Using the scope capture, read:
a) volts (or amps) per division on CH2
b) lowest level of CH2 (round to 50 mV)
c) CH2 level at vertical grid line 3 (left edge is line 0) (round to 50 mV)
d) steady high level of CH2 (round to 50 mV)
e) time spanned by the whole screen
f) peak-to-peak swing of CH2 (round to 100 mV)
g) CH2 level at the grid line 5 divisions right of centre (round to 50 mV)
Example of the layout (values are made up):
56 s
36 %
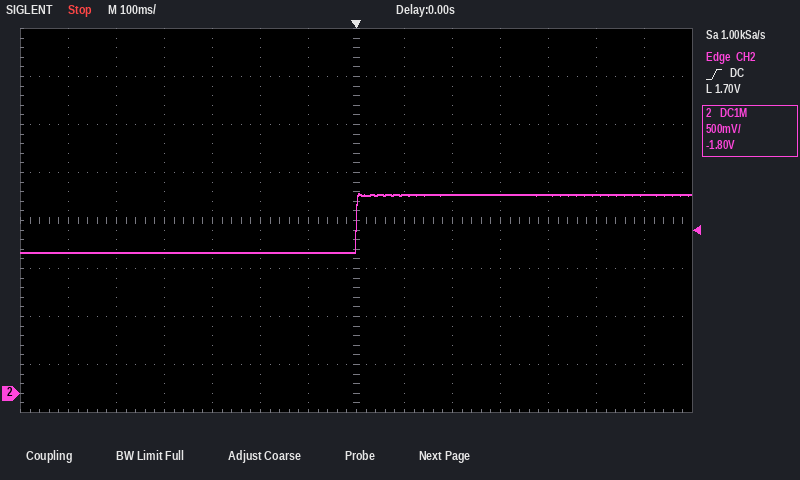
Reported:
500 mV
1.45 V
1.45 V
2.05 V
1.4 s
600 mV
2.05 V
